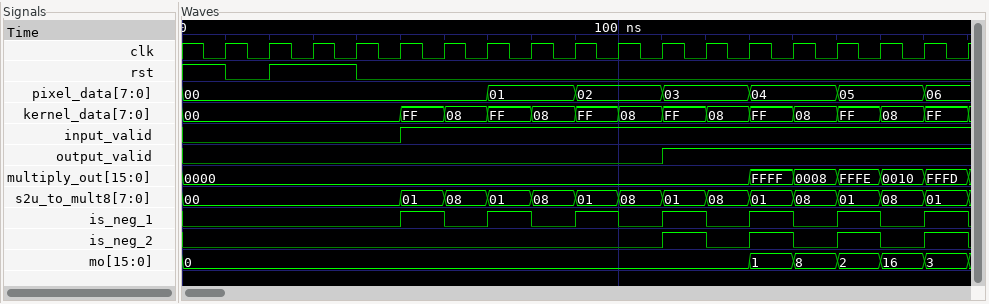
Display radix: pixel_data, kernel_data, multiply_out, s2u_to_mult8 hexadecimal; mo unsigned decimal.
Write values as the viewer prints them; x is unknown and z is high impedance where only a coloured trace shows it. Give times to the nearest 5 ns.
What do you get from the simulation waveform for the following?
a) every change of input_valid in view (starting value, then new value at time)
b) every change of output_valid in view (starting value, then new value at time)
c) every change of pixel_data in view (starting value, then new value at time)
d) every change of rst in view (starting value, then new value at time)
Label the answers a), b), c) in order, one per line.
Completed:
a) 0, 1 at 50 ns
b) 0, 1 at 110 ns
c) 00, 01 at 70 ns, 02 at 90 ns, 03 at 110 ns, 04 at 130 ns, 05 at 150 ns, 06 at 170 ns
d) 1, 0 at 10 ns, 1 at 20 ns, 0 at 40 ns
